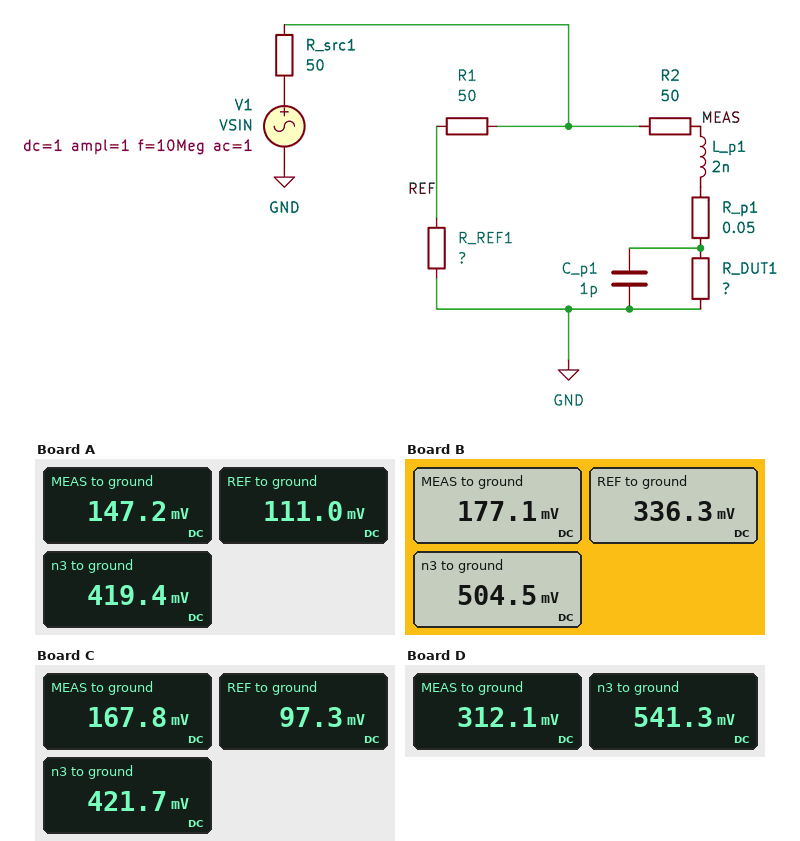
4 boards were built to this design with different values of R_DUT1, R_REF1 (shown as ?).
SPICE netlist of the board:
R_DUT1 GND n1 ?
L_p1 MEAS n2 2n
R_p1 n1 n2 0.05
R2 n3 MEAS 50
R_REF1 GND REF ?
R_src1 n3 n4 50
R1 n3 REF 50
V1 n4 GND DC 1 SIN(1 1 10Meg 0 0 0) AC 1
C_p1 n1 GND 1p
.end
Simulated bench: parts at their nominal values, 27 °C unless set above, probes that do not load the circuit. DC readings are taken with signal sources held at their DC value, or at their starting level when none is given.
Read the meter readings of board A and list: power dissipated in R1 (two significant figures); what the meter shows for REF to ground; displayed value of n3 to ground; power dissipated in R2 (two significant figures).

1.9 mW
111.0 mV
419.4 mV
1.5 mW
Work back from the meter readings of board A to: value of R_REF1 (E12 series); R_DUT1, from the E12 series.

18 Ω
27 Ω
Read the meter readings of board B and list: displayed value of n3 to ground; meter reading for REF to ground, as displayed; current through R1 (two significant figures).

504.5 mV
336.3 mV
3.4 mA
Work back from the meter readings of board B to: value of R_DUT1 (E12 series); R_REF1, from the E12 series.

27 Ω
100 Ω
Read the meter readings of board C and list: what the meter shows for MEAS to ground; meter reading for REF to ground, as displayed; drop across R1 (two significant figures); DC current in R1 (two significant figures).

167.8 mV
97.3 mV
320 mV
6.5 mA
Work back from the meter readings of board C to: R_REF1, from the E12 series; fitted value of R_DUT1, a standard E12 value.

15 Ω
33 Ω
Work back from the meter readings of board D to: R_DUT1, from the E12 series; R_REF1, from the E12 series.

68 Ω
68 Ω
